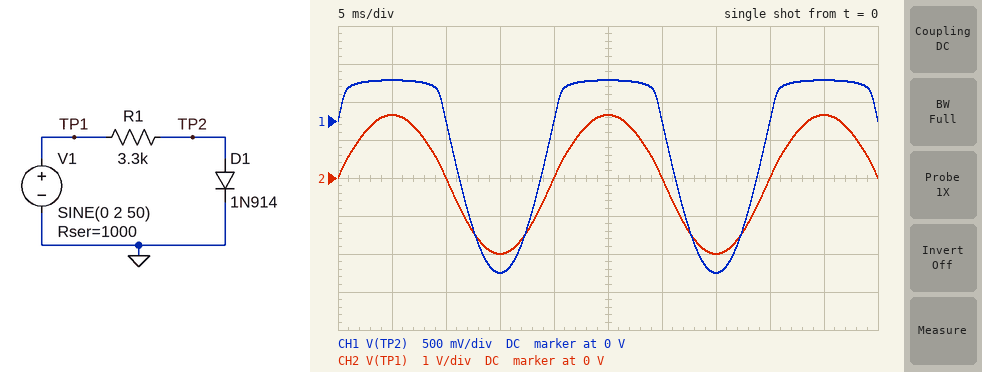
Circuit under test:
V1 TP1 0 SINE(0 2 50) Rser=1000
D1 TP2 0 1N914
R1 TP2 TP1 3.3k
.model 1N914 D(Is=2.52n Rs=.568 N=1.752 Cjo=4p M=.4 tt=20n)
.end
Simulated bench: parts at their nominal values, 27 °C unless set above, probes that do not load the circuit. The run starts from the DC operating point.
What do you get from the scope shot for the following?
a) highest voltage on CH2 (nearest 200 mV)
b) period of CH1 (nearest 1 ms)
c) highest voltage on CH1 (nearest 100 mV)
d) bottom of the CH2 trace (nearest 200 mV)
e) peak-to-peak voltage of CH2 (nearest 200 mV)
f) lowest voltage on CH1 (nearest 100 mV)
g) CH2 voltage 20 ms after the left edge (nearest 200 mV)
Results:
1.6 V
20 ms
500 mV
-2.0 V
3.6 V
-2.0 V
0 V
